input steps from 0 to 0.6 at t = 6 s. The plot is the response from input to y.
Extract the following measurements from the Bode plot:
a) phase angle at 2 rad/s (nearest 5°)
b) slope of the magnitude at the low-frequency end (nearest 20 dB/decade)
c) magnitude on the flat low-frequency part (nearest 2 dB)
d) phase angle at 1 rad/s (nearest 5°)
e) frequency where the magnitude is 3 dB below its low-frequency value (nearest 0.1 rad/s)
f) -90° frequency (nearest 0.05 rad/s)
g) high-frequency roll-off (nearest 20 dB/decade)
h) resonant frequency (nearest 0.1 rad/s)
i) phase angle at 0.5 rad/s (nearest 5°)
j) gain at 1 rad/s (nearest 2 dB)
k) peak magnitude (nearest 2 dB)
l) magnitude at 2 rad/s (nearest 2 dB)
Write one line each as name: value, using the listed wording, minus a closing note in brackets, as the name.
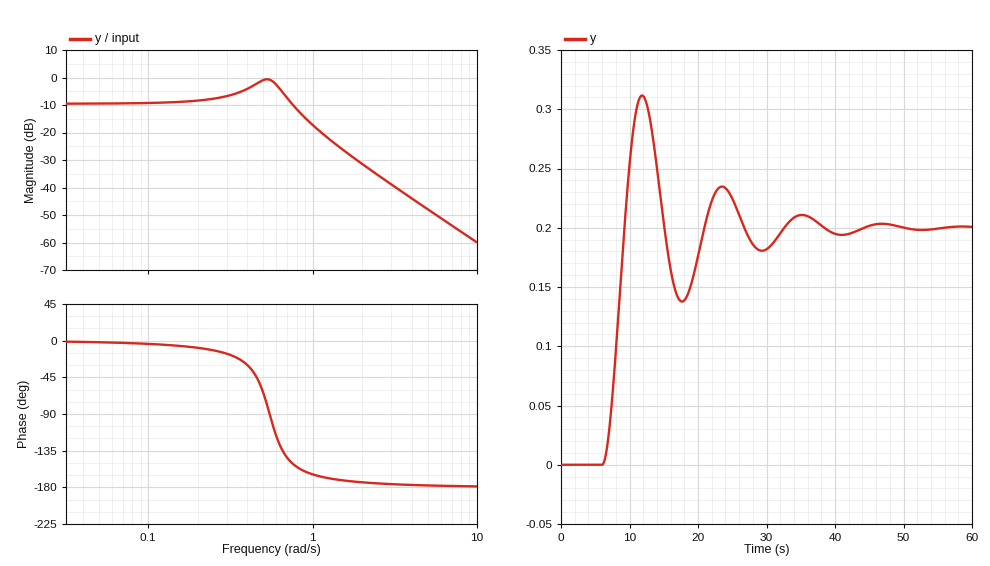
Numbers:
phase angle at 2 rad/s: -175°
slope of the magnitude at the low-frequency end: 0 dB/decade
magnitude on the flat low-frequency part: -10 dB
phase angle at 1 rad/s: -165°
frequency where the magnitude is 3 dB below its low-frequency value: 0.8 rad/s
-90° frequency: 0.55 rad/s
high-frequency roll-off: -40 dB/decade
resonant frequency: 0.5 rad/s
phase angle at 0.5 rad/s: -65°
gain at 1 rad/s: -18 dB
peak magnitude: 0 dB
magnitude at 2 rad/s: -32 dB
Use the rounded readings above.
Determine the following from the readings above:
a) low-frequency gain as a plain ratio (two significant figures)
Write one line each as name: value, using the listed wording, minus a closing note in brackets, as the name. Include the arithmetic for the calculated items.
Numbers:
low-frequency gain as a plain ratio: 10^(-10 / 20) = 0.32
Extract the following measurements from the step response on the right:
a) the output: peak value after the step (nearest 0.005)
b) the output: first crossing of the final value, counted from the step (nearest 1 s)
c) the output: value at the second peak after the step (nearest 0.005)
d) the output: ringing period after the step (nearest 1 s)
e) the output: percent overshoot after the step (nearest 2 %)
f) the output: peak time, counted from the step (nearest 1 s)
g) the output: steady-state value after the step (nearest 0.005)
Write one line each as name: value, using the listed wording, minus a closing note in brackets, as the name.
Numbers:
the output: peak value after the step: 0.310
the output: first crossing of the final value, counted from the step: 3 s
the output: value at the second peak after the step: 0.235
the output: ringing period after the step: 12 s
the output: percent overshoot after the step: 56 %
the output: peak time, counted from the step: 6 s
the output: steady-state value after the step: 0.200
